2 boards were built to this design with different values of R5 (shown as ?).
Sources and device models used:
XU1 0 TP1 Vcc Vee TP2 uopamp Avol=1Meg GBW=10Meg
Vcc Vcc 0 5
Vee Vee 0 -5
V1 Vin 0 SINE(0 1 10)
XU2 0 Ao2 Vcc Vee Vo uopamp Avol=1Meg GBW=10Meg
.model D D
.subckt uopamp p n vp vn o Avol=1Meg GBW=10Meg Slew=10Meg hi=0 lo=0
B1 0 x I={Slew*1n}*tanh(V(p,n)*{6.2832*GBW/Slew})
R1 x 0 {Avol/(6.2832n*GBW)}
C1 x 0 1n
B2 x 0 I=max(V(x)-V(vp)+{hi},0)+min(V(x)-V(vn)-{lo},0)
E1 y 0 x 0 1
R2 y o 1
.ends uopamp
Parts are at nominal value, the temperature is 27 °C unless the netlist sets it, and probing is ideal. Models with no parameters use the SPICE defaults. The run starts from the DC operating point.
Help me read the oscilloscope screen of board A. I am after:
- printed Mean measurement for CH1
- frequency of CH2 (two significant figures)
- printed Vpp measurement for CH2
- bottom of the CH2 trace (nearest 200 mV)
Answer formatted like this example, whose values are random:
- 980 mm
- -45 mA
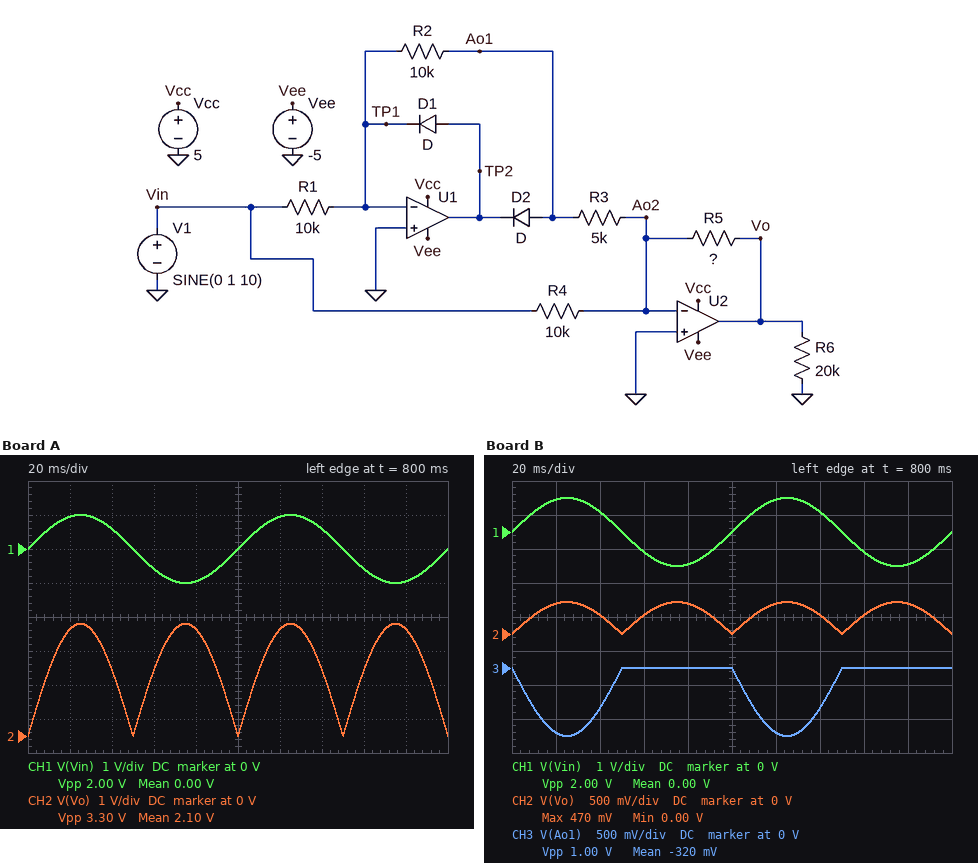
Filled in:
- 0.00 V
- 20 Hz
- 3.30 V
- 0 V
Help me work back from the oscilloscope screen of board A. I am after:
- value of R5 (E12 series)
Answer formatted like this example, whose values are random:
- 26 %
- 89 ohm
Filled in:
- 33 kΩ
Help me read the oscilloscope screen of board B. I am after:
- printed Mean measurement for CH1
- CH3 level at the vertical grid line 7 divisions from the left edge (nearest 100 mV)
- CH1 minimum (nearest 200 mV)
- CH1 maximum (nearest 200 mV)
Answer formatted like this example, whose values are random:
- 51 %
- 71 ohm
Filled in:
- 0.00 V
- -600 mV
- -1.0 V
- 1.0 V
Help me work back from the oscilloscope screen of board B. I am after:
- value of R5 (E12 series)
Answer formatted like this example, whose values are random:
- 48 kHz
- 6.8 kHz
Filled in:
- 4.7 kΩ
